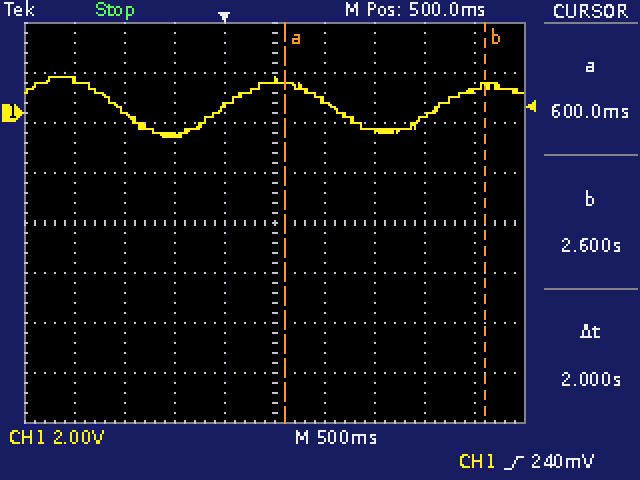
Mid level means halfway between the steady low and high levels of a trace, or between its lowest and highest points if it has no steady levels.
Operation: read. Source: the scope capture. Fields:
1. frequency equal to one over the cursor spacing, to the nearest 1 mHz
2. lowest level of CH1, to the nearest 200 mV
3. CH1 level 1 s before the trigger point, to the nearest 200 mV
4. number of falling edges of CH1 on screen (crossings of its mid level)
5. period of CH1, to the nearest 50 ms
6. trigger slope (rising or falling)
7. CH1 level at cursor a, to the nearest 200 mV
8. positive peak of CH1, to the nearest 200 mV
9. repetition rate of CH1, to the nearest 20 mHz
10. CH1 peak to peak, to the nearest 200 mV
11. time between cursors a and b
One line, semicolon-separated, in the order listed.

500 mHz; -1.0 V; 0.0 V; 2; 2.15 s; rising; 1.2 V; 1.4 V; 460 mHz; 2.4 V; 2 s
